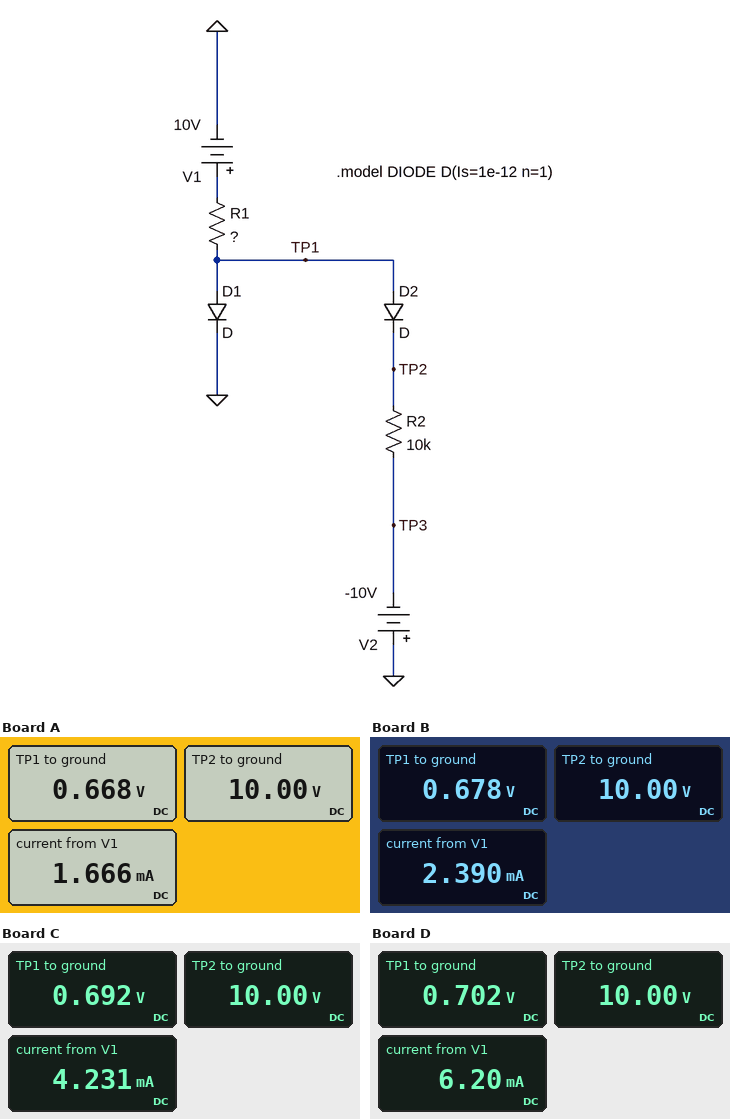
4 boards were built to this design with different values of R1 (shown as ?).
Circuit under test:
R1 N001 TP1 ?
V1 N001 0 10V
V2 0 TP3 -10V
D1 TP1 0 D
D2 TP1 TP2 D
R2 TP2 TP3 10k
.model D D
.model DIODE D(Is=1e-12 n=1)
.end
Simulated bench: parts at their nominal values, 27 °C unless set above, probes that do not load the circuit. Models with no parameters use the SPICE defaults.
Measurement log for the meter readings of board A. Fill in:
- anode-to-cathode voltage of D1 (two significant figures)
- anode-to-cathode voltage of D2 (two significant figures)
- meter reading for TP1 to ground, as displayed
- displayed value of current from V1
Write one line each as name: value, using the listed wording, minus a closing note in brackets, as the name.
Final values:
anode-to-cathode voltage of D1: 670 mV
anode-to-cathode voltage of D2: -9.3 V
meter reading for TP1 to ground, as displayed: 0.668 V
displayed value of current from V1: 1.666 mA
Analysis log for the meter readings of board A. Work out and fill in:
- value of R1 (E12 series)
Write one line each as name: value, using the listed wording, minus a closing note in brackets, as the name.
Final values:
value of R1: 5.6 kΩ
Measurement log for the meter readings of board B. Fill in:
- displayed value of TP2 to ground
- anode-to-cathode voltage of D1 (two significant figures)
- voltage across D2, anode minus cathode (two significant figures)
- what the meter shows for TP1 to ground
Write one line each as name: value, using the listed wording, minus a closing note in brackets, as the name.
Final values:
displayed value of TP2 to ground: 10.00 V
anode-to-cathode voltage of D1: 680 mV
voltage across D2, anode minus cathode: -9.3 V
what the meter shows for TP1 to ground: 0.678 V
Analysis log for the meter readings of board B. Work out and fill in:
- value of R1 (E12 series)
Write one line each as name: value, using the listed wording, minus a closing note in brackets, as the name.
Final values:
value of R1: 3.9 kΩ
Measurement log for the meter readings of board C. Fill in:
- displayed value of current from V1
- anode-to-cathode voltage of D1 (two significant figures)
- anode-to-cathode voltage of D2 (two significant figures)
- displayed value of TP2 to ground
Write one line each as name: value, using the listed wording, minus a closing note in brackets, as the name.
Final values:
displayed value of current from V1: 4.231 mA
anode-to-cathode voltage of D1: 690 mV
anode-to-cathode voltage of D2: -9.3 V
displayed value of TP2 to ground: 10.00 V
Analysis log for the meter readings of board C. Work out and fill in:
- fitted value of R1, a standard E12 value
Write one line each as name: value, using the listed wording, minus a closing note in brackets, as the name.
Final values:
fitted value of R1, a standard E12 value: 2.2 kΩ
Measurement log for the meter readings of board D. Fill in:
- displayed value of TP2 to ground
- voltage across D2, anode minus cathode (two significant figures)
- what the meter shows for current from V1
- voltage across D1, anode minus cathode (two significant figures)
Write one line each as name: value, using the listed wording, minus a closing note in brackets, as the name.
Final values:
displayed value of TP2 to ground: 10.00 V
voltage across D2, anode minus cathode: -9.3 V
what the meter shows for current from V1: 6.20 mA
voltage across D1, anode minus cathode: 700 mV
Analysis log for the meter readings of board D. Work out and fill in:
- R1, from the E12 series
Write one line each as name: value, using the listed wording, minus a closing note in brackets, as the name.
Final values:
R1, from the E12 series: 1.5 kΩ
